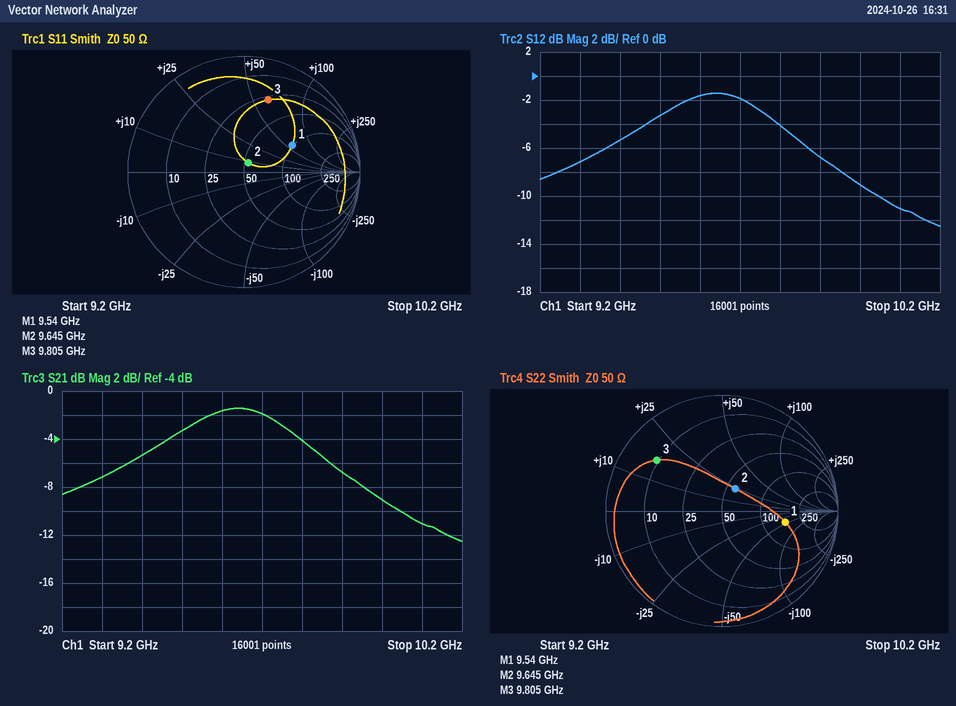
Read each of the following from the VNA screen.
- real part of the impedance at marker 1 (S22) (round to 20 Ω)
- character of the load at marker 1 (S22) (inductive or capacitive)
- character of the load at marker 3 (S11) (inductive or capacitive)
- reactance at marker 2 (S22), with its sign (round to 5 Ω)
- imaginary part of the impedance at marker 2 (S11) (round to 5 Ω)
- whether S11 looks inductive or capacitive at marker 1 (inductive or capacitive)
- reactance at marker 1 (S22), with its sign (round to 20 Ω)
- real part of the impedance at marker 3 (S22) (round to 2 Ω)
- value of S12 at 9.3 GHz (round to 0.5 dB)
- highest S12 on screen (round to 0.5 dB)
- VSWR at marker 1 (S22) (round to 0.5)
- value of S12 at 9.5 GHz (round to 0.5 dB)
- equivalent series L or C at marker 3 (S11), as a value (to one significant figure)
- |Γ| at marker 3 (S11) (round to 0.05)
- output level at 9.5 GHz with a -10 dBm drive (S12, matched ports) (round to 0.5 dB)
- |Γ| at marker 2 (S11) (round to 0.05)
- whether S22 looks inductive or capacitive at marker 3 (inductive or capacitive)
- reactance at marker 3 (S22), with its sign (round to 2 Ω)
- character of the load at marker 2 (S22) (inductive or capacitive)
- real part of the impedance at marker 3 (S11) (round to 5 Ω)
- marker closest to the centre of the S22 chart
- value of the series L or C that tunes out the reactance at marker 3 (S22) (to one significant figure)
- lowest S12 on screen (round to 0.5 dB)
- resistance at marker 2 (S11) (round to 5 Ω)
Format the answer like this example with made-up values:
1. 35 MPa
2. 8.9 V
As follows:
1. 160 Ω
2. capacitive
3. inductive
4. +25 Ω
5. +10 Ω
6. inductive
7. -40 Ω
8. 10 Ω
9. -7.0 dB
10. -1.5 dB
11. 3.5
12. -3.5 dB
13. 1.0 nH
14. 0.65
15. -13.5 dBm
16. 0.10
17. inductive
18. +16 Ω
19. inductive
20. 30 Ω
21. marker 2
22. 1.0 pF
23. -12.5 dB
24. 55 Ω
